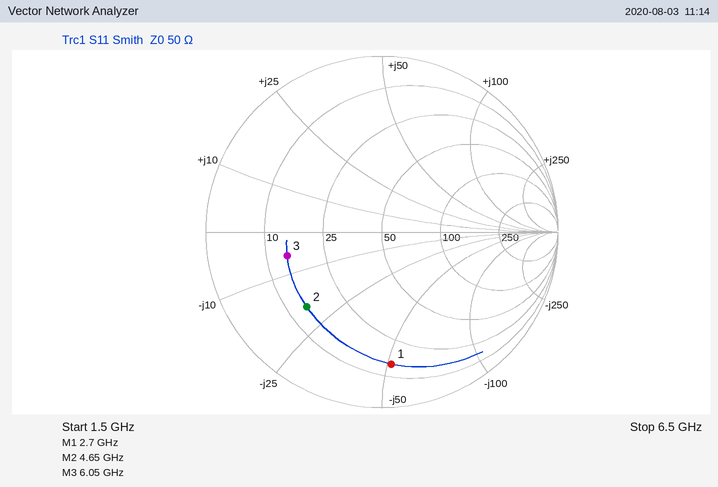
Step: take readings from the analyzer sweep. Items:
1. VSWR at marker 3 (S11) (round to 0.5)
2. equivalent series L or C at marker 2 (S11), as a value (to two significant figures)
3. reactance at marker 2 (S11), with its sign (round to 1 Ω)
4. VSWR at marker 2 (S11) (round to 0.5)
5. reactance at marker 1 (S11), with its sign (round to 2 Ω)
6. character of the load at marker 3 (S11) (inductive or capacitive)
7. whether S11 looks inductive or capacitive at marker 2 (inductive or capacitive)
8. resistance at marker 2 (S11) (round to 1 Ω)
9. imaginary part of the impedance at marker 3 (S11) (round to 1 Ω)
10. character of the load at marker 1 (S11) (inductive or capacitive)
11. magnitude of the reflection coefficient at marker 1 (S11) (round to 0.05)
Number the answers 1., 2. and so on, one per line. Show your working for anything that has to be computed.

1. 3.5
2. C = 1/(2π × 4.65 GHz × 19 Ω) ≈ 1.8 pF
3. -19 Ω
4. 4.0
5. -52 Ω
6. capacitive
7. capacitive
8. 14 Ω
9. -6 Ω
10. capacitive
11. 0.75
